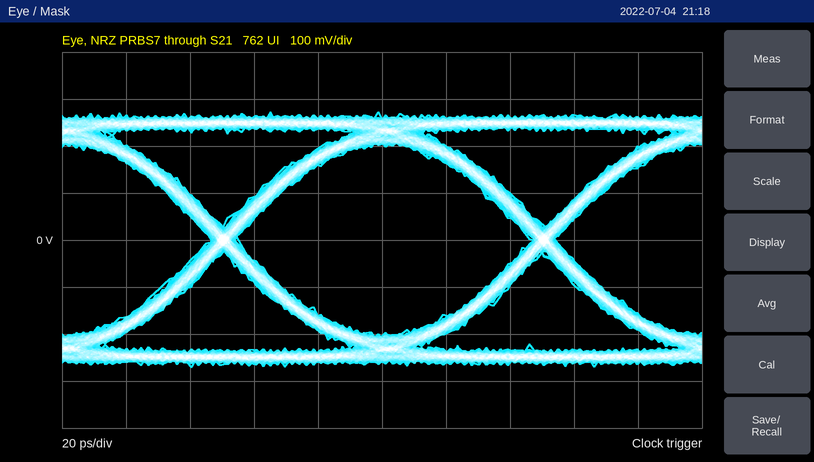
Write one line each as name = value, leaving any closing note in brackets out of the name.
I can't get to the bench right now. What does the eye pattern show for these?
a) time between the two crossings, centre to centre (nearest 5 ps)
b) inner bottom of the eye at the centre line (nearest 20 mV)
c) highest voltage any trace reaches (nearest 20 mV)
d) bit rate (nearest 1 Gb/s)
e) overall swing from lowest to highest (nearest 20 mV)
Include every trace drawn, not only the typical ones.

time between the two crossings, centre to centre = 100 ps
inner bottom of the eye at the centre line = -200 mV
highest voltage any trace reaches = 280 mV
bit rate = 10 Gb/s
overall swing from lowest to highest = 540 mV
